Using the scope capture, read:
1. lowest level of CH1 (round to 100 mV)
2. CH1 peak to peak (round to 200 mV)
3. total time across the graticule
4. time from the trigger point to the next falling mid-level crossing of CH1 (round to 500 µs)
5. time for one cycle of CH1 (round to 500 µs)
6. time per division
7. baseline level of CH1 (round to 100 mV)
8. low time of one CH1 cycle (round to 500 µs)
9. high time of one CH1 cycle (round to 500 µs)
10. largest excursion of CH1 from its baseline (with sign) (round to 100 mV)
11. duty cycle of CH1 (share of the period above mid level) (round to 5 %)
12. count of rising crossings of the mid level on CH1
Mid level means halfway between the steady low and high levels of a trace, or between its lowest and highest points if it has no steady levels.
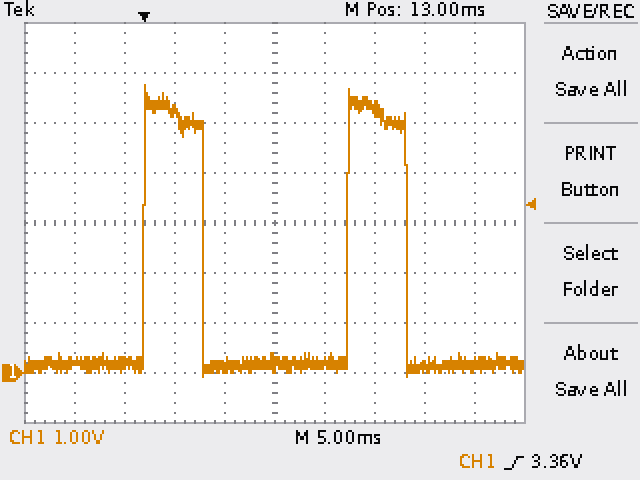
-100 mV
5.8 V
50 ms
6.0 ms
20.5 ms
5 ms
200 mV
14.5 ms
6.0 ms
+5.6 V
30 %
2
